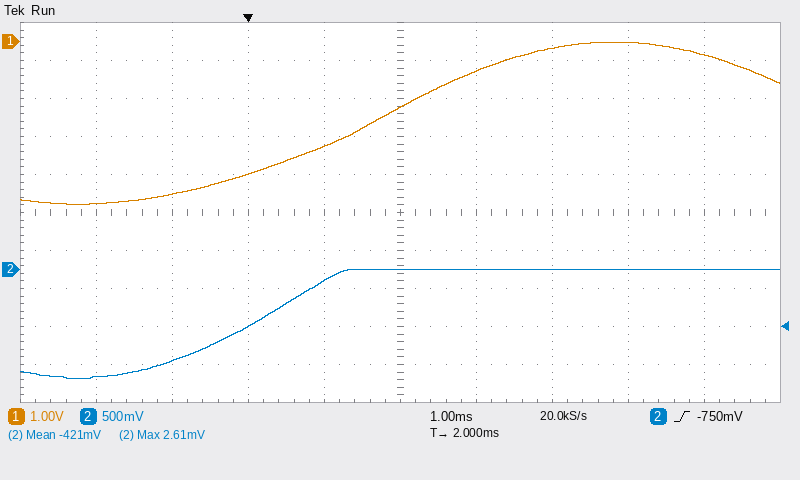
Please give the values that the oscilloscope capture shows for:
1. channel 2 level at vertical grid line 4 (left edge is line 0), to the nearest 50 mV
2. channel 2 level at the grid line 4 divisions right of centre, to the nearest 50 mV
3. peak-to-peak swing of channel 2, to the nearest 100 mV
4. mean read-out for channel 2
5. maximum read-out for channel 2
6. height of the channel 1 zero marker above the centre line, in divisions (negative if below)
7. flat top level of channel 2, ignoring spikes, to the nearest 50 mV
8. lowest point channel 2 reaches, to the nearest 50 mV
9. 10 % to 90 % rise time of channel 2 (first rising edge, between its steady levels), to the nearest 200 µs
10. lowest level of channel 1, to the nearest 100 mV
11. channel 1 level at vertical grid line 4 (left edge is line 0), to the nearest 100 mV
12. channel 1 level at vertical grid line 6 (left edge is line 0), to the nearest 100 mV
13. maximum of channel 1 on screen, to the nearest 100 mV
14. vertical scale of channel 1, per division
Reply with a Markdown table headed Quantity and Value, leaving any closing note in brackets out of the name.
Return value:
| Quantity | Value |
|---|---|
| channel 2 level at vertical grid line 4 (left edge is line 0), to the nearest 50 mV | -150 mV |
| channel 2 level at the grid line 4 divisions right of centre, to the nearest 50 mV | 0 mV |
| peak-to-peak swing of channel 2, to the nearest 100 mV | 1.40 V |
| mean read-out for channel 2 | -421 mV |
| maximum read-out for channel 2 | 2.61 mV |
| height of the channel 1 zero marker above the centre line, in divisions | +4.5 div |
| flat top level of channel 2, ignoring spikes, to the nearest 50 mV | 0 mV |
| lowest point channel 2 reaches, to the nearest 50 mV | -1.45 V |
| 10 % to 90 % rise time of channel 2 (first rising edge, between its steady levels), to the nearest 200 µs | 2.2 ms |
| lowest level of channel 1, to the nearest 100 mV | -4.3 V |
| channel 1 level at vertical grid line 4 (left edge is line 0), to the nearest 100 mV | -2.8 V |
| channel 1 level at vertical grid line 6 (left edge is line 0), to the nearest 100 mV | -800 mV |
| maximum of channel 1 on screen, to the nearest 100 mV | 0.0 V |
| vertical scale of channel 1, per division | 1 V |
